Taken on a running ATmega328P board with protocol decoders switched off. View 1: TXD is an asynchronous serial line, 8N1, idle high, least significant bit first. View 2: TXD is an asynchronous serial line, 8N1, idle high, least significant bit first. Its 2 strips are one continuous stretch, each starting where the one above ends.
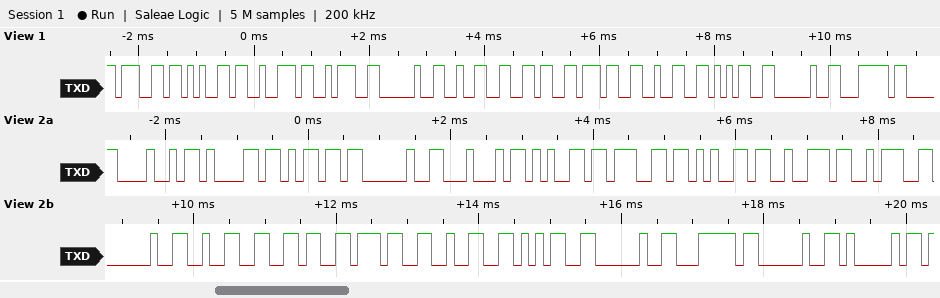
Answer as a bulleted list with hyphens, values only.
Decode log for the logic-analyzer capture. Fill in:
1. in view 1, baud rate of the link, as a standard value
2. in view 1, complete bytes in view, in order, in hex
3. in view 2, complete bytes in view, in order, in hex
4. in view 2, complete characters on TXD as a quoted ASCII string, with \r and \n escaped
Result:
- 9600 baud
- 67 65 72 3A 20 32 36 37 32 35 20 7C
- 48 61 6D 20 44 65 67 65 72 3A 20 32 36 37 32 35 20 7C 20 41
- "Ham Deger: 26725 | A"
